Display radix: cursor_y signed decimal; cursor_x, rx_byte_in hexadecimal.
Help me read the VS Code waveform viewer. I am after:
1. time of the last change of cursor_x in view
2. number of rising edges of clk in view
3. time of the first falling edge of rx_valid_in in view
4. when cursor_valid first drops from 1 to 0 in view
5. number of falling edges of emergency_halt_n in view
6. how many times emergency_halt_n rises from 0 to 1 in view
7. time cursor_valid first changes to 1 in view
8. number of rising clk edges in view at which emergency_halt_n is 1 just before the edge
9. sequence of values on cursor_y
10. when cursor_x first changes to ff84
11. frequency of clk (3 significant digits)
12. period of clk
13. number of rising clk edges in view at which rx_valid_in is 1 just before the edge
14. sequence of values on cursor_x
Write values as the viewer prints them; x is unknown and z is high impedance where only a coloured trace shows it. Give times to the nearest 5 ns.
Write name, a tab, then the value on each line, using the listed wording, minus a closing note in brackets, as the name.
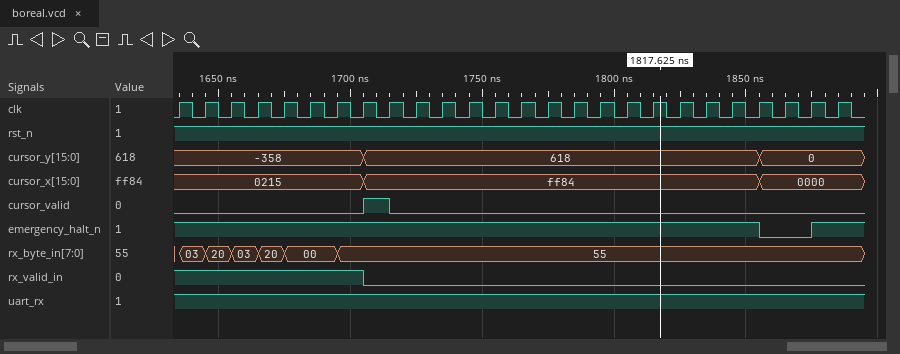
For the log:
time of the last change of cursor_x in view	1855 ns
number of rising edges of clk in view	26
time of the first falling edge of rx_valid_in in view	1705 ns
when cursor_valid first drops from 1 to 0 in view	1715 ns
number of falling edges of emergency_halt_n in view	1
how many times emergency_halt_n rises from 0 to 1 in view	1
time cursor_valid first changes to 1 in view	1705 ns
number of rising clk edges in view at which emergency_halt_n is 1 just before the edge	24
sequence of values on cursor_y	-358, 618, 0
when cursor_x first changes to ff84	1705 ns
frequency of clk	100 MHz
period of clk	10 ns
number of rising clk edges in view at which rx_valid_in is 1 just before the edge	8
sequence of values on cursor_x	0215, ff84, 0000
